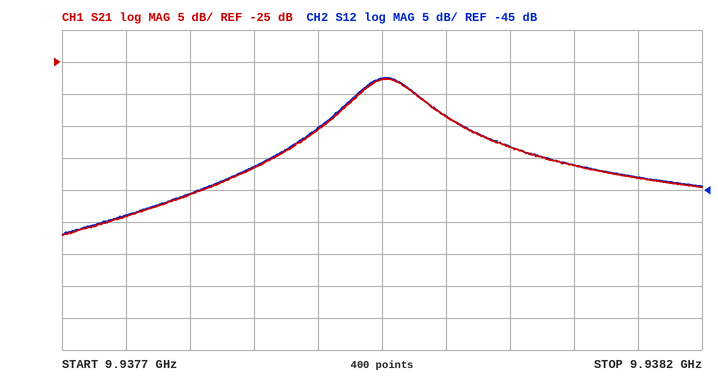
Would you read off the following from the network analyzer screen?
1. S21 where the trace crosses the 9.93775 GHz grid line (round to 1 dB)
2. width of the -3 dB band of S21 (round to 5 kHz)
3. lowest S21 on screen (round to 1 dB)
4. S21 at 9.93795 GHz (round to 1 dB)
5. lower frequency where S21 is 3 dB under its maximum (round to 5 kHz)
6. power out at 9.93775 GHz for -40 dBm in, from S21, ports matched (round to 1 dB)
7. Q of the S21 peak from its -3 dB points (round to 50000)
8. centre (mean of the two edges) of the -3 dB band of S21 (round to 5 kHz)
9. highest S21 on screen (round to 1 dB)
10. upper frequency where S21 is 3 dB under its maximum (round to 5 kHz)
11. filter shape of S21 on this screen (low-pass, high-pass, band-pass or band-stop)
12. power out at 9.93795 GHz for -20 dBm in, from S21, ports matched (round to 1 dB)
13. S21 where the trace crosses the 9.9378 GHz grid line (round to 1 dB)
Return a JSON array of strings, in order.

["-49 dB", "50 kHz", "-52 dB", "-28 dB", "9.937930 GHz", "-89 dBm", "200000", "9.937955 GHz", "-28 dB", "9.937980 GHz", "band-pass", "-48 dBm", "-46 dB"]
